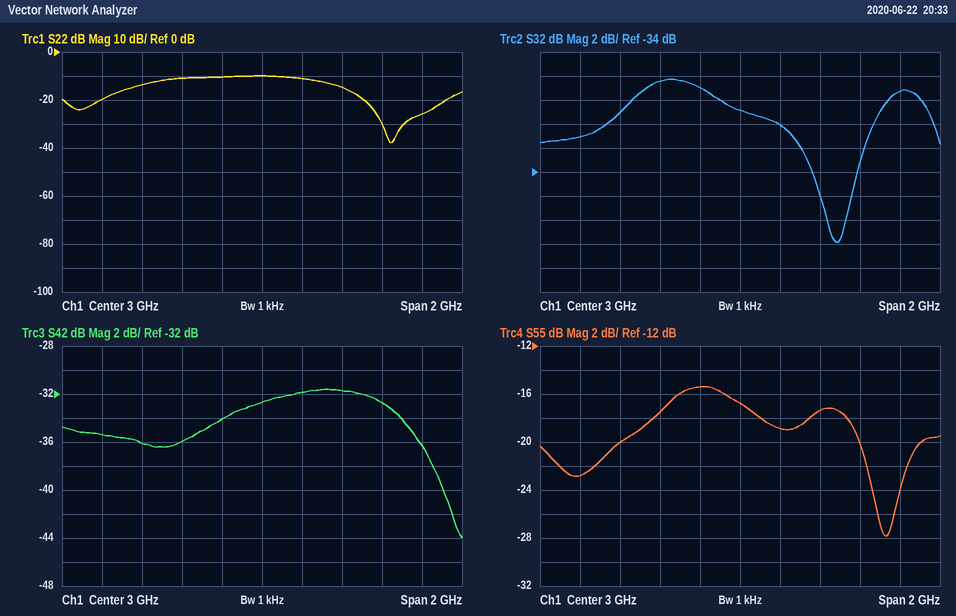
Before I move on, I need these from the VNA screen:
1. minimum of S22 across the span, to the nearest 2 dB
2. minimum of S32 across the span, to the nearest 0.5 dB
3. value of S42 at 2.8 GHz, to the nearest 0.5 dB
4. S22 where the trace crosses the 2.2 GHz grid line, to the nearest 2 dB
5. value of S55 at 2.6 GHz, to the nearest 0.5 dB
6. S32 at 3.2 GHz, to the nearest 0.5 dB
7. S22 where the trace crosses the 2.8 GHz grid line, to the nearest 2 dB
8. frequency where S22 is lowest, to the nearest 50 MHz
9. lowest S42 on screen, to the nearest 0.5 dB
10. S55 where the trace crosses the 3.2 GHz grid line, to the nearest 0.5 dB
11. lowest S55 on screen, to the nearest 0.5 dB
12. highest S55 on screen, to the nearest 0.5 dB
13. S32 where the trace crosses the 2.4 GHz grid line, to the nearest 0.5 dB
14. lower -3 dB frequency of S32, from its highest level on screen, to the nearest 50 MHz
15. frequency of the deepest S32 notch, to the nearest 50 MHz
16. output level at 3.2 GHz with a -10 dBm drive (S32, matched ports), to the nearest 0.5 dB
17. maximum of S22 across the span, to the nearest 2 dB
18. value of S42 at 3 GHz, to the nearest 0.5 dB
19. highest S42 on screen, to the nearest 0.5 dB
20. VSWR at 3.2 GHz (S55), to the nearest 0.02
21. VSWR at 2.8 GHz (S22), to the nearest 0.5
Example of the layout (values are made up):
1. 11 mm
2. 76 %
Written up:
1. -38 dB
2. -40.0 dB
3. -34.0 dB
4. -20 dB
5. -17.5 dB
6. -30.0 dB
7. -10 dB
8. 3.65 GHz
9. -44.0 dB
10. -19.0 dB
11. -28.0 dB
12. -15.5 dB
13. -29.0 dB
14. 2.40 GHz
15. 3.50 GHz
16. -40.0 dBm
17. -10 dB
18. -32.5 dB
19. -31.5 dB
20. 1.26
21. 2.0
